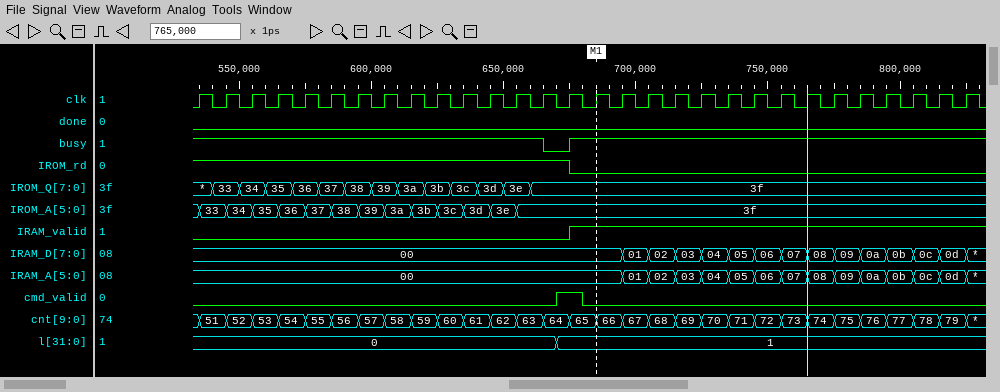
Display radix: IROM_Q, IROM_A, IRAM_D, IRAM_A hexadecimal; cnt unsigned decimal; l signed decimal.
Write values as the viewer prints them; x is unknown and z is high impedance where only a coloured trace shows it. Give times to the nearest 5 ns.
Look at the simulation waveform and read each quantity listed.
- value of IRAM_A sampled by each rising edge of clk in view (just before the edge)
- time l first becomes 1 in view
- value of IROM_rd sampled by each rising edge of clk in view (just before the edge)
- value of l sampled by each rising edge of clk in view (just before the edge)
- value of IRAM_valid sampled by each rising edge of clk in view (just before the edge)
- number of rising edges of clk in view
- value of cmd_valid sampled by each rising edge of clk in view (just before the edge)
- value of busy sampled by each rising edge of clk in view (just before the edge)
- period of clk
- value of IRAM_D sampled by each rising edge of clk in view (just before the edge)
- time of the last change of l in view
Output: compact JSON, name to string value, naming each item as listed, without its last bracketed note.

{"value of IRAM_A sampled by each rising edge of clk in view": "00, 00, 00, 00, 00, 00, 00, 00, 00, 00, 00, 00, 00, 00, 00, 00, 00, 01, 02, 03, 04, 05, 06, 07, 08, 09, 0a, 0b, 0c, 0d", "time l first becomes 1 in view": "670 ns", "value of IROM_rd sampled by each rising edge of clk in view": "1 1 1 1 1 1 1 1 1 1 1 1 1 1 1 0 0 0 0 0 0 0 0 0 0 0 0 0 0 0", "value of l sampled by each rising edge of clk in view": "0, 0, 0, 0, 0, 0, 0, 0, 0, 0, 0, 0, 0, 0, 1, 1, 1, 1, 1, 1, 1, 1, 1, 1, 1, 1, 1, 1, 1, 1", "value of IRAM_valid sampled by each rising edge of clk in view": "0 0 0 0 0 0 0 0 0 0 0 0 0 0 0 1 1 1 1 1 1 1 1 1 1 1 1 1 1 1", "number of rising edges of clk in view": "30", "value of cmd_valid sampled by each rising edge of clk in view": "0 0 0 0 0 0 0 0 0 0 0 0 0 0 1 0 0 0 0 0 0 0 0 0 0 0 0 0 0 0", "value of busy sampled by each rising edge of clk in view": "1 1 1 1 1 1 1 1 1 1 1 1 1 1 0 1 1 1 1 1 1 1 1 1 1 1 1 1 1 1", "period of clk": "10 ns", "value of IRAM_D sampled by each rising edge of clk in view": "00, 00, 00, 00, 00, 00, 00, 00, 00, 00, 00, 00, 00, 00, 00, 00, 00, 01, 02, 03, 04, 05, 06, 07, 08, 09, 0a, 0b, 0c, 0d", "time of the last change of l in view": "670 ns"}
